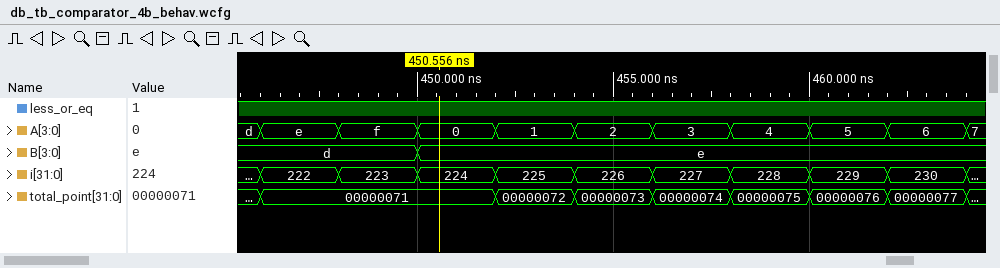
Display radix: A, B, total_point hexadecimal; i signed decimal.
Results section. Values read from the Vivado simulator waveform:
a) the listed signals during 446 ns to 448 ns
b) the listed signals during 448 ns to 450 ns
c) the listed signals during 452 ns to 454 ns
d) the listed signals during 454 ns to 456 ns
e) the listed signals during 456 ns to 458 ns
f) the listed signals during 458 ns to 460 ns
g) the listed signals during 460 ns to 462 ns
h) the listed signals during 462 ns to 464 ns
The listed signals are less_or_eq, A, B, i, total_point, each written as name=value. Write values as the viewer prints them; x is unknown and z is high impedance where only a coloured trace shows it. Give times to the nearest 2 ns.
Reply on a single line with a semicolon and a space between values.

less_or_eq=1, A=e, B=d, i=222, total_point=00000071; less_or_eq=1, A=f, B=d, i=223, total_point=00000071; less_or_eq=1, A=1, B=e, i=225, total_point=00000072; less_or_eq=1, A=2, B=e, i=226, total_point=00000073; less_or_eq=1, A=3, B=e, i=227, total_point=00000074; less_or_eq=1, A=4, B=e, i=228, total_point=00000075; less_or_eq=1, A=5, B=e, i=229, total_point=00000076; less_or_eq=1, A=6, B=e, i=230, total_point=00000077
